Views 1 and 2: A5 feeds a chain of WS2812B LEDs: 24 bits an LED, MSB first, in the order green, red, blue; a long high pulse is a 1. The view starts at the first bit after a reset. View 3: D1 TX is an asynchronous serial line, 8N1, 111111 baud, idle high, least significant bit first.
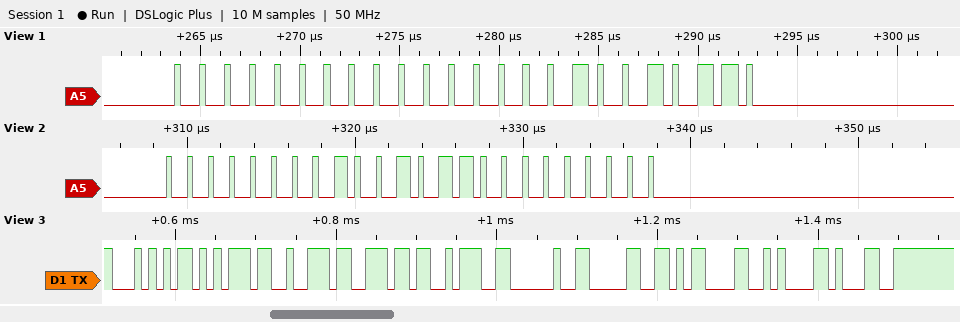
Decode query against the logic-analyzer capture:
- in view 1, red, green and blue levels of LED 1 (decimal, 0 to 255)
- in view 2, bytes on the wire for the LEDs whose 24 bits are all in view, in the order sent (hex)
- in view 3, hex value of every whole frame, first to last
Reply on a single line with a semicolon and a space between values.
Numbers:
0, 0, 150; 00 96 00; 0x54 0x75 0x72 0x6E 0x3A 0x20 0x30 0x0D 0x0A 0x31
